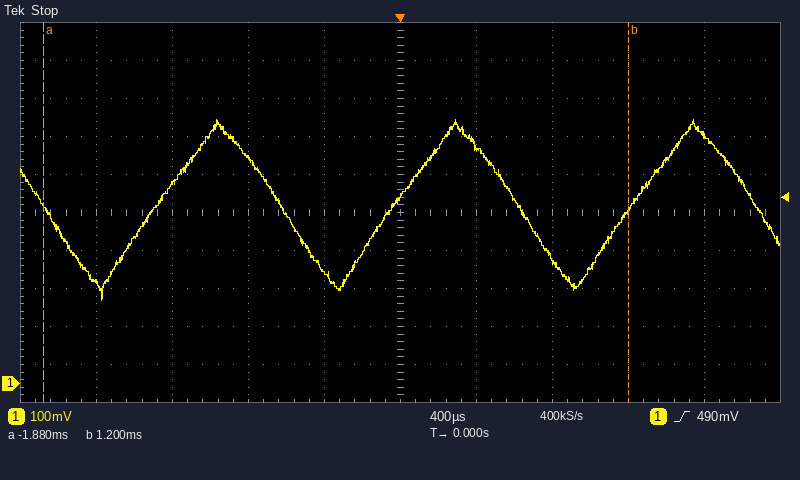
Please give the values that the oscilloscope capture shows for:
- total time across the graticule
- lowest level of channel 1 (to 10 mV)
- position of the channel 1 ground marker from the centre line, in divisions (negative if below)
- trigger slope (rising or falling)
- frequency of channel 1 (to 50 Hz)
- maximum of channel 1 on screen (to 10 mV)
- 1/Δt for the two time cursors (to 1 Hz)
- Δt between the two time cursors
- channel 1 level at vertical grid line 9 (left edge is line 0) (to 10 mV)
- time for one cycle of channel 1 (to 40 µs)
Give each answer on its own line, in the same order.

4 ms
220 mV
-4.5 div
rising
800 Hz
690 mV
325 Hz
3.08 ms
650 mV
1.24 ms
